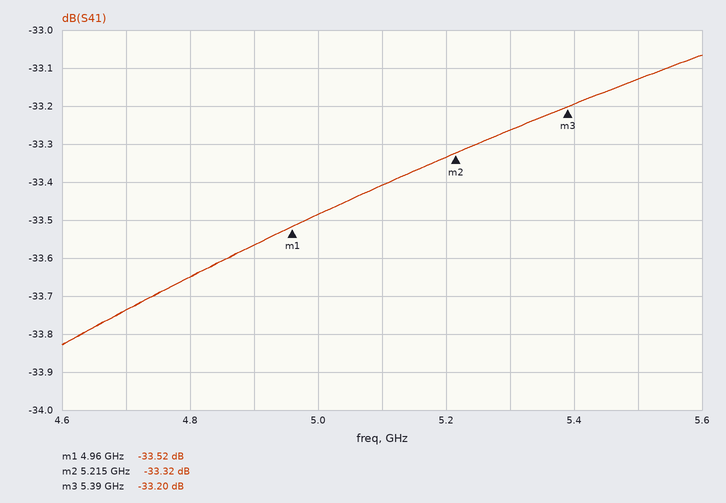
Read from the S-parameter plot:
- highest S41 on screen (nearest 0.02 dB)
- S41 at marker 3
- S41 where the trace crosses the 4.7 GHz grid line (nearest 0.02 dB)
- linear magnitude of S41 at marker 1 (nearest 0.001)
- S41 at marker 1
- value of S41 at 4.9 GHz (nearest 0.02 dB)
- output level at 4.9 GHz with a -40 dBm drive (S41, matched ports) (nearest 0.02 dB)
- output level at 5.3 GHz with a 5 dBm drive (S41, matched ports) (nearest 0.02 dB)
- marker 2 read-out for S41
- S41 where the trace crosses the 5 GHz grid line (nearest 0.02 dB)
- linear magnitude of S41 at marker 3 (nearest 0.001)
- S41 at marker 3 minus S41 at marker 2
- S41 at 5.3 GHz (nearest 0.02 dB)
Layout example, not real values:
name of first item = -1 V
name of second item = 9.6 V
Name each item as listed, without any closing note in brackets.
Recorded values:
highest S41 on screen = -33.06 dB
S41 at marker 3 = -33.20 dB
S41 where the trace crosses the 4.7 GHz grid line = -33.74 dB
linear magnitude of S41 at marker 1 = 0.021
S41 at marker 1 = -33.52 dB
value of S41 at 4.9 GHz = -33.56 dB
output level at 4.9 GHz with a -40 dBm drive (S41, matched ports) = -73.56 dBm
output level at 5.3 GHz with a 5 dBm drive (S41, matched ports) = -28.26 dBm
marker 2 read-out for S41 = -33.32 dB
S41 where the trace crosses the 5 GHz grid line = -33.48 dB
linear magnitude of S41 at marker 3 = 0.022
S41 at marker 3 minus S41 at marker 2 = 0.12 dB
S41 at 5.3 GHz = -33.26 dB
